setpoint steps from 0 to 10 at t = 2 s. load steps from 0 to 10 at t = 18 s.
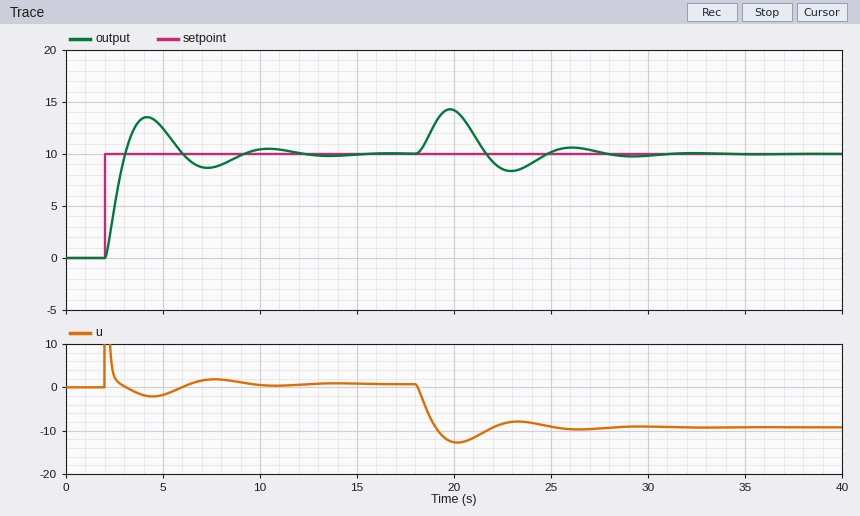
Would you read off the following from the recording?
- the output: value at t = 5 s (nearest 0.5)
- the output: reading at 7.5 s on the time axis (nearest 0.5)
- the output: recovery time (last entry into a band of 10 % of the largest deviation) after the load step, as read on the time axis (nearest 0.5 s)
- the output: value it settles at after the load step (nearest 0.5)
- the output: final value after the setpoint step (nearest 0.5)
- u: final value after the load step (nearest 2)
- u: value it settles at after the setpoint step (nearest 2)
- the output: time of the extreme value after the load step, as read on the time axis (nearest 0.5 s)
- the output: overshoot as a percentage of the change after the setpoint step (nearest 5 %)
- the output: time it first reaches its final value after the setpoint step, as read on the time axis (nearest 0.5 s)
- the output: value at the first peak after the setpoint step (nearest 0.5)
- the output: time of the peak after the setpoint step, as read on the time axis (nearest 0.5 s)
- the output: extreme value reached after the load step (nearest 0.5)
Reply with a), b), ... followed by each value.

a) 12.5
b) 8.5
c) 27.0 s
d) 10.0
e) 10.0
f) -10
g) 0
h) 20.0 s
i) 35 %
j) 3.0 s
k) 13.5
l) 4.0 s
m) 14.5
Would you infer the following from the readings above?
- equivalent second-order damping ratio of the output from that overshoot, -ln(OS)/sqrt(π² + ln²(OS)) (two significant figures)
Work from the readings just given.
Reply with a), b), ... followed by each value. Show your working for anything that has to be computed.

a) ln(0.35) = -1.050; 1.050 / sqrt(9.870 + 1.102) = 0.32
